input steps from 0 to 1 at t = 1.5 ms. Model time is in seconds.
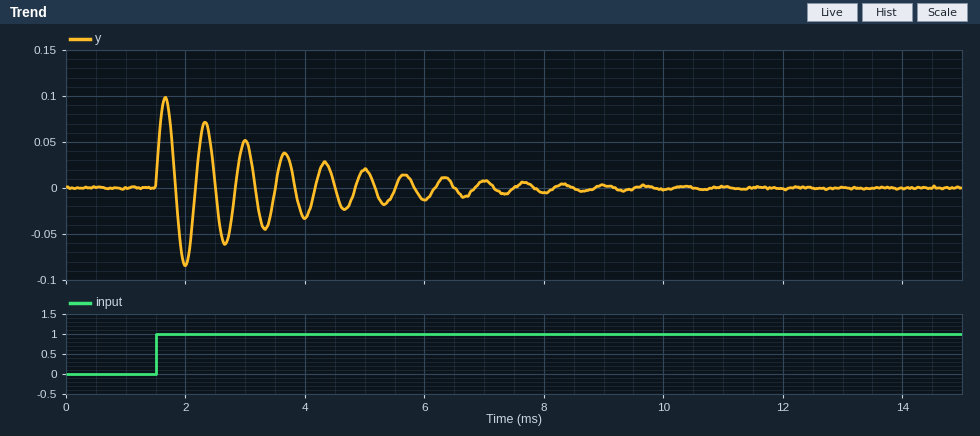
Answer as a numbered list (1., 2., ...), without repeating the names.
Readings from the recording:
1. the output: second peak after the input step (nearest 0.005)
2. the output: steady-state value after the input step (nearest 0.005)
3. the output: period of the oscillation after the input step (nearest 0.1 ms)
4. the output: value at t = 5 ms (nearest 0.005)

1. 0.070
2. 0.000
3. 0.7 ms
4. 0.020
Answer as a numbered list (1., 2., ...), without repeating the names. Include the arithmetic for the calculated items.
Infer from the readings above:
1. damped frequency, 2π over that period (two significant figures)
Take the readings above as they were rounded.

1. 2π / 0.7 = 9.0 rad/ms
